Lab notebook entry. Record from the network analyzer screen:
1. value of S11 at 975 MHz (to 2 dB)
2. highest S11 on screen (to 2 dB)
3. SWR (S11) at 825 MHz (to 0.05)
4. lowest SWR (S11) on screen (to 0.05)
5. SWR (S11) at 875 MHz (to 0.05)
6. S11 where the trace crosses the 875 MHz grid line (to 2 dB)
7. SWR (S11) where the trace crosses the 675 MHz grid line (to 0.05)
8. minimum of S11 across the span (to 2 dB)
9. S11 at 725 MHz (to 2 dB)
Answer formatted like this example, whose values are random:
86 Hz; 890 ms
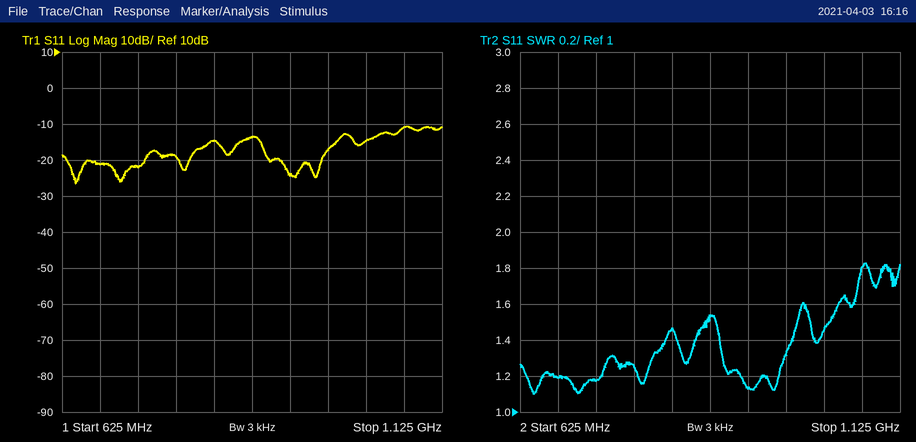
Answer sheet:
-18 dB; -10 dB; 1.45; 1.10; 1.55; -14 dB; 1.20; -26 dB; -22 dB
